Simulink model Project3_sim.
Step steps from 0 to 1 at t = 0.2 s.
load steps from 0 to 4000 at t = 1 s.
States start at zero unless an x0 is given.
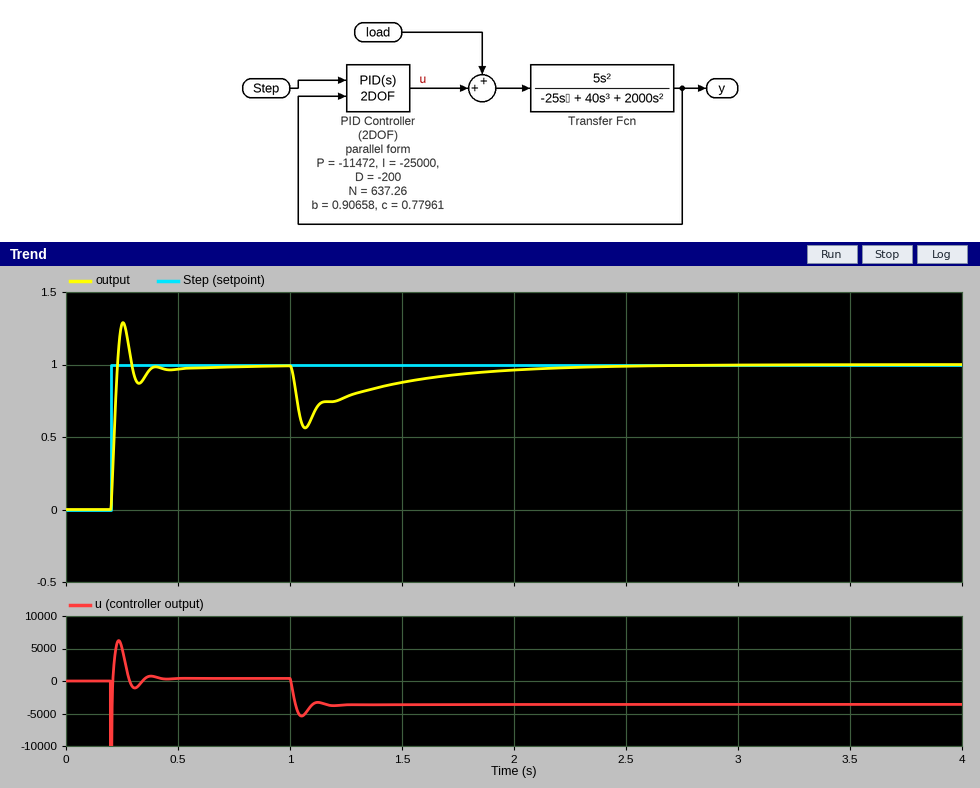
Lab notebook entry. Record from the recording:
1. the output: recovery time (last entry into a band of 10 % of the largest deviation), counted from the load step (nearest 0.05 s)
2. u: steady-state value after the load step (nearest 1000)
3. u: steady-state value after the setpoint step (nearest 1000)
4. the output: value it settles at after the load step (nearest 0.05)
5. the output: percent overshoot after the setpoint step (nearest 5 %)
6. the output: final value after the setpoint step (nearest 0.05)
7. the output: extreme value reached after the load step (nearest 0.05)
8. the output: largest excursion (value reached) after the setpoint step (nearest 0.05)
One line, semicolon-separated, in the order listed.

0.95 s; -4000; 0; 1.00; 30 %; 1.00; 0.55; 1.30
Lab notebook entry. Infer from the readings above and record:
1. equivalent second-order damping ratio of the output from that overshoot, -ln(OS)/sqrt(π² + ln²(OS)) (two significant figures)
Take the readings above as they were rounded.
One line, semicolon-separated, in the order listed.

0.36
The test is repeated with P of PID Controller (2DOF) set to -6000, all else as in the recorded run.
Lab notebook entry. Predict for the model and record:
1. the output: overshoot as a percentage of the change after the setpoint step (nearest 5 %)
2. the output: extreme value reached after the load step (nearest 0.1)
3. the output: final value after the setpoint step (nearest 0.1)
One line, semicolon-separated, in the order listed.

25 %; 0.3; 1.0
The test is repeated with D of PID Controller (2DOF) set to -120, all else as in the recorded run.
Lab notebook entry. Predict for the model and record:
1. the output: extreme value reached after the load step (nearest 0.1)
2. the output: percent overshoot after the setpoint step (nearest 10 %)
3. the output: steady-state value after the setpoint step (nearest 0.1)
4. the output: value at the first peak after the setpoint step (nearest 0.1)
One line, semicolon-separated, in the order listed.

0.5; 50 %; 1.0; 1.5
